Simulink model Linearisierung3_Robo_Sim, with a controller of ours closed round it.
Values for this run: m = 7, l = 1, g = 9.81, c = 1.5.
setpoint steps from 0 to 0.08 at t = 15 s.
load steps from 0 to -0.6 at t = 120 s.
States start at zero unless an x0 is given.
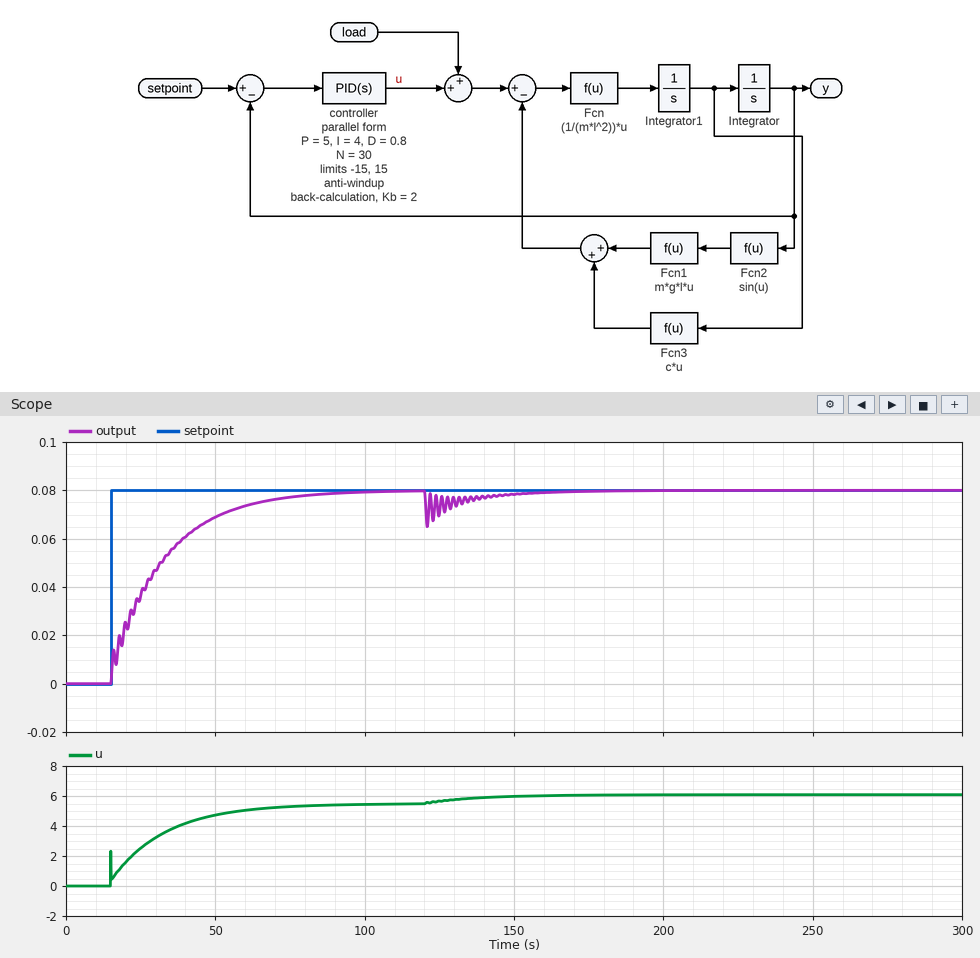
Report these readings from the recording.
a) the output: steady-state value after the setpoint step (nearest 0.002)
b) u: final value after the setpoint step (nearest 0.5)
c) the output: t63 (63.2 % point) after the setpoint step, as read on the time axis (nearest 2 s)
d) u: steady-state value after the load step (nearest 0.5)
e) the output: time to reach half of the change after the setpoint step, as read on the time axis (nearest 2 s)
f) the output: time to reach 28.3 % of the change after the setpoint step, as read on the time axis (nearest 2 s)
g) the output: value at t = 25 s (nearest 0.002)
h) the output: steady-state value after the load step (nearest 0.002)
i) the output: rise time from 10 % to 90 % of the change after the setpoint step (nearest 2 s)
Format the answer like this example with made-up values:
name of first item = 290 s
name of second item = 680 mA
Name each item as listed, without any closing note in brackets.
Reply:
the output: steady-state value after the setpoint step = 0.080
u: final value after the setpoint step = 5.5
the output: t63 (63.2 % point) after the setpoint step, as read on the time axis = 32 s
u: steady-state value after the load step = 6.0
the output: time to reach half of the change after the setpoint step, as read on the time axis = 26 s
the output: time to reach 28.3 % of the change after the setpoint step, as read on the time axis = 20 s
the output: value at t = 25 s = 0.036
the output: steady-state value after the load step = 0.080
the output: rise time from 10 % to 90 % of the change after the setpoint step = 40 s
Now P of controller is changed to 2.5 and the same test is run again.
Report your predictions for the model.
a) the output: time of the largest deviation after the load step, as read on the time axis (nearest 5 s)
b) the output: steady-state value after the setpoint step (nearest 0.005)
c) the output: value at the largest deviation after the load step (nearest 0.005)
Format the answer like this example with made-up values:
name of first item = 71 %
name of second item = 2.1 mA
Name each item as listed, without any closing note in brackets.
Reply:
the output: time of the largest deviation after the load step, as read on the time axis = 120 s
the output: steady-state value after the setpoint step = 0.080
the output: value at the largest deviation after the load step = 0.065
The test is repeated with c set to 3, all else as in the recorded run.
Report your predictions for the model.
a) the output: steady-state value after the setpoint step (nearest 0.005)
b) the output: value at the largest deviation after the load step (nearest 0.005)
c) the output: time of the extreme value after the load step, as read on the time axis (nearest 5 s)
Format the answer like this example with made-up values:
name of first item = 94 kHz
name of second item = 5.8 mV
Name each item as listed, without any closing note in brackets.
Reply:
the output: steady-state value after the setpoint step = 0.080
the output: value at the largest deviation after the load step = 0.065
the output: time of the extreme value after the load step, as read on the time axis = 120 s
